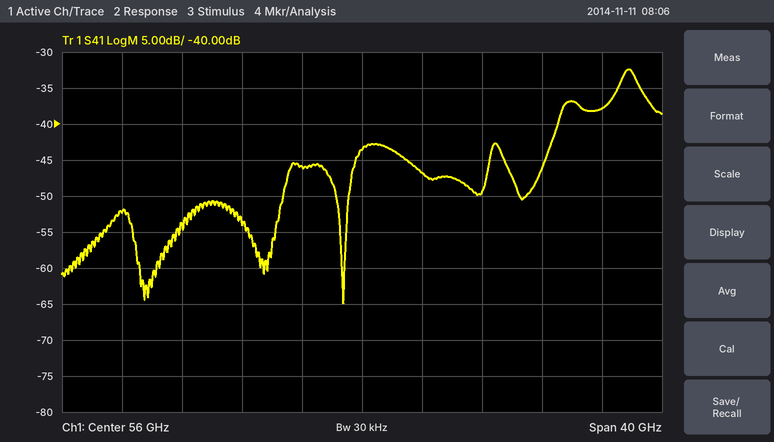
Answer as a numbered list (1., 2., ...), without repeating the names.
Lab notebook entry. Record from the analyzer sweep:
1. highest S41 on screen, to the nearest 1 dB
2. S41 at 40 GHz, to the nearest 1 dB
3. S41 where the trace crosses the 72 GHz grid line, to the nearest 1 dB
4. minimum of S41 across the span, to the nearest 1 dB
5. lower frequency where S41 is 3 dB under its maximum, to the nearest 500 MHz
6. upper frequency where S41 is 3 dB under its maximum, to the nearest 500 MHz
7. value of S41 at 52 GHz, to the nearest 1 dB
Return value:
1. -32 dB
2. -52 dB
3. -38 dB
4. -65 dB
5. 73.0 GHz
6. 74.5 GHz
7. -46 dB
